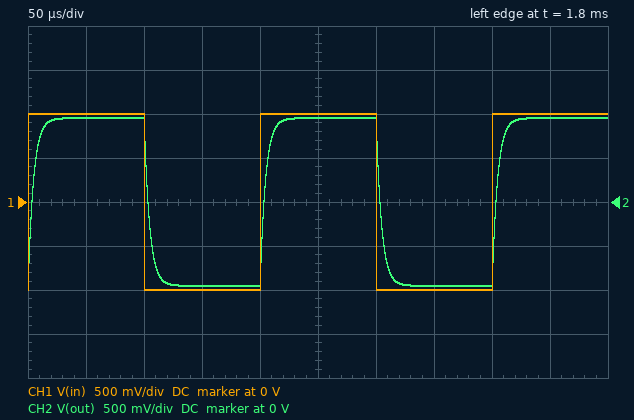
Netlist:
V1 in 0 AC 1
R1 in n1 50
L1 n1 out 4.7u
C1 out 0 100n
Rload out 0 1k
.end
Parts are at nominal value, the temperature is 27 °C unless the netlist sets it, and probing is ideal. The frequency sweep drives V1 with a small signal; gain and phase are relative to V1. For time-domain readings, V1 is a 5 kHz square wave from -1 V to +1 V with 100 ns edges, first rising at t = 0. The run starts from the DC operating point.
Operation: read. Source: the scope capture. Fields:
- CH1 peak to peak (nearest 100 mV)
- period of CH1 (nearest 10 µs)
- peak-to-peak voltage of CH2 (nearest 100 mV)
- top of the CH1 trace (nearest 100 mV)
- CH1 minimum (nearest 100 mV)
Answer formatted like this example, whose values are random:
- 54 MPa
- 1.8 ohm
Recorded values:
- 2.0 V
- 200 µs
- 1.9 V
- 1.0 V
- -1.0 V
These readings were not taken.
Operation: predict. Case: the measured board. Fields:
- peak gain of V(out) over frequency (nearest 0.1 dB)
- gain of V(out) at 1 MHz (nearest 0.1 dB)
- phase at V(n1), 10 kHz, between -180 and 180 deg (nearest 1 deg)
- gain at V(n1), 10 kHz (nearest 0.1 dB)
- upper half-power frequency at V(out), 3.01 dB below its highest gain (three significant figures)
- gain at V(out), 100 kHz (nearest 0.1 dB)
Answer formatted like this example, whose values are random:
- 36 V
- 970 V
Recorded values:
- -0.4 dB
- -31.1 dB
- -17 deg
- -0.8 dB
- 34.1 kHz
- -10.3 dB
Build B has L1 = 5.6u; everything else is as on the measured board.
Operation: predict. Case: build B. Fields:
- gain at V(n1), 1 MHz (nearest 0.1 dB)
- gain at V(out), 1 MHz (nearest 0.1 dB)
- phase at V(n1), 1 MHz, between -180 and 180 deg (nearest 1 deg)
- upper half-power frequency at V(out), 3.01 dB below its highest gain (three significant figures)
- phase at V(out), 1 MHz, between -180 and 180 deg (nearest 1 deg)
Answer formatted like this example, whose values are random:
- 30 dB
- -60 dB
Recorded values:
- -5.1 dB
- -31.6 dB
- 56 deg
- 34.2 kHz
- -124 deg
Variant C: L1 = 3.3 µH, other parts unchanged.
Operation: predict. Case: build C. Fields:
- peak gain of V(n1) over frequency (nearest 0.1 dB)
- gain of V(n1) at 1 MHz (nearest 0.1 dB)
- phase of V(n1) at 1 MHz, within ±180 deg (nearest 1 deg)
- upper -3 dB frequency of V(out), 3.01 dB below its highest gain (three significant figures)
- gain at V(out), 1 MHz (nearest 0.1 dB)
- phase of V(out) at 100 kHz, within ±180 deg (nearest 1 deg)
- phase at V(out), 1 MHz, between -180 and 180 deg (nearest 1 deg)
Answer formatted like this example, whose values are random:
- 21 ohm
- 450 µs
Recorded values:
- 0 dB
- -8.9 dB
- 69 deg
- 33.9 kHz
- -30.5 dB
- -74 deg
- -111 deg
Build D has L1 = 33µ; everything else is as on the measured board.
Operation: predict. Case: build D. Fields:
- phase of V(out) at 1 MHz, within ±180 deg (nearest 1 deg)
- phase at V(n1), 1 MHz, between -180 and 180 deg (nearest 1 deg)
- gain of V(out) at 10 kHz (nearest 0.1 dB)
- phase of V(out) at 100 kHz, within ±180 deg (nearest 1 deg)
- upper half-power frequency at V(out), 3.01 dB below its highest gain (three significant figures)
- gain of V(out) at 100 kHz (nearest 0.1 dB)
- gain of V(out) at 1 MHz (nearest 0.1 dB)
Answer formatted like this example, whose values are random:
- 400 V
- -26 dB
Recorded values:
- -166 deg
- 14 deg
- -0.7 dB
- -95 deg
- 38.3 kHz
- -10.0 dB
- -42.5 dB
